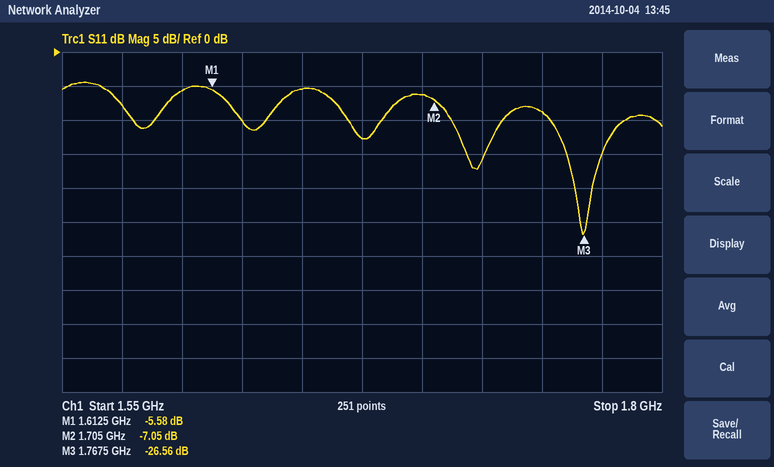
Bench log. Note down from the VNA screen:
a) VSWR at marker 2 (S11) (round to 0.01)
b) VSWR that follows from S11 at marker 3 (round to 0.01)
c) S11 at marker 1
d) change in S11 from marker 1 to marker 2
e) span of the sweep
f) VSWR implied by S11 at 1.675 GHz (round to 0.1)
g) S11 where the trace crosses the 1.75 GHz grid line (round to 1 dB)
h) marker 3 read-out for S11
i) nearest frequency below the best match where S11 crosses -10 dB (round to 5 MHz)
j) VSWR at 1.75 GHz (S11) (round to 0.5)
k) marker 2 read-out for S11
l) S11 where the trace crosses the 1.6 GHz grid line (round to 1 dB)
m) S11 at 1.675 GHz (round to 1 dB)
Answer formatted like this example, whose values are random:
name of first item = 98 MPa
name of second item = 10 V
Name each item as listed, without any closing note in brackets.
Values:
VSWR at marker 2 (S11) = 2.60
VSWR that follows from S11 at marker 3 = 1.10
S11 at marker 1 = -5.58 dB
change in S11 from marker 1 to marker 2 = -1.47 dB
span of the sweep = 250 MHz
VSWR implied by S11 at 1.675 GHz = 1.6
S11 where the trace crosses the 1.75 GHz grid line = -9 dB
marker 3 read-out for S11 = -26.56 dB
nearest frequency below the best match where S11 crosses -10 dB = 1.755 GHz
VSWR at 1.75 GHz (S11) = 2.0
marker 2 read-out for S11 = -7.05 dB
S11 where the trace crosses the 1.6 GHz grid line = -6 dB
S11 at 1.675 GHz = -13 dB
